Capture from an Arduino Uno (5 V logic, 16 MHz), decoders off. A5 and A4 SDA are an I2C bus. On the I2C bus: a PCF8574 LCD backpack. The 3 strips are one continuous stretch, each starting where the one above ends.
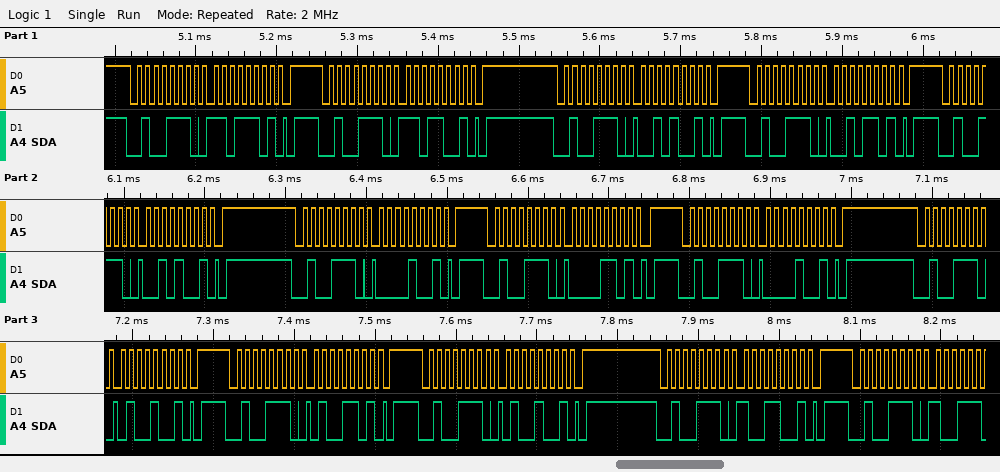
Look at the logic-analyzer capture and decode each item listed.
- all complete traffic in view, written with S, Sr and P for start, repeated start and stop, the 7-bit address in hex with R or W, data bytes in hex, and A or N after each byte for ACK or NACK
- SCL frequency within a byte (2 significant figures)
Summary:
S 27W A DD A P S 27W A D9 A P S 27W A 29 A P S 27W A 2D A P S 27W A 29 A P S 27W A 09 A P S 27W A 0D A P S 27W A 09 A P S 27W A 49 A P S 27W A 4D A P S 27W A 49 A P S 27W A 99 A P S 27W A
100 kHz
